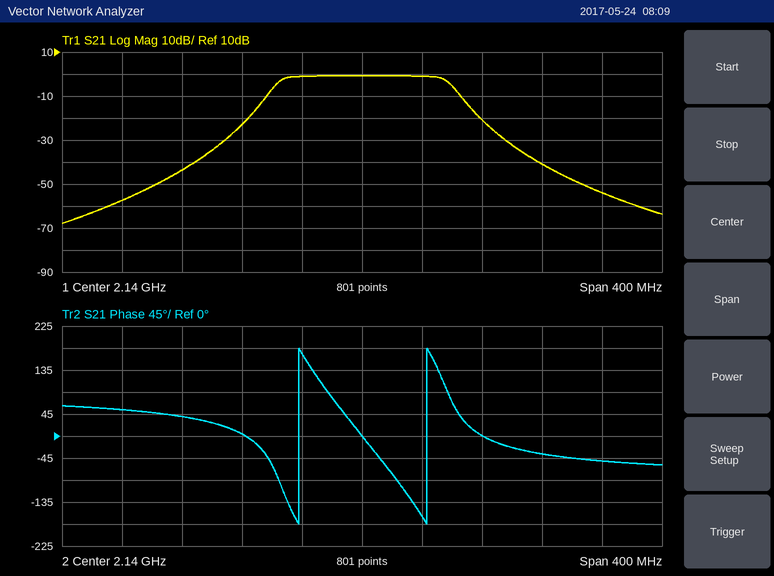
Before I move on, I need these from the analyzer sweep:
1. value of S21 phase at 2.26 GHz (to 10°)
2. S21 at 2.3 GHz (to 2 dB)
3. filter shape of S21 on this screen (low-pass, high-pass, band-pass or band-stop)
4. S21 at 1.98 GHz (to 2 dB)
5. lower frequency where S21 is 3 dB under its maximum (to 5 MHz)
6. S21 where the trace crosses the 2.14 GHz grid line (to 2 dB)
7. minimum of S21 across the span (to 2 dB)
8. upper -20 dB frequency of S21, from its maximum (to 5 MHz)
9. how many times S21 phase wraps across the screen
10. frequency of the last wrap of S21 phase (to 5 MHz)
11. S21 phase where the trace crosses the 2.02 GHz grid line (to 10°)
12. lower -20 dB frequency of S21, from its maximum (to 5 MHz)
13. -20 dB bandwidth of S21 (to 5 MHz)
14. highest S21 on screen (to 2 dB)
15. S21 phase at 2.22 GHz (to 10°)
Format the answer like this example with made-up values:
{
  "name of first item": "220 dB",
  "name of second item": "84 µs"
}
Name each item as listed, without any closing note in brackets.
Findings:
{
  "value of S21 phase at 2.26 GHz": "-40°",
  "S21 at 2.3 GHz": "-54 dB",
  "filter shape of S21 on this screen": "band-pass",
  "S21 at 1.98 GHz": "-58 dB",
  "lower frequency where S21 is 3 dB under its maximum": "2.085 GHz",
  "S21 where the trace crosses the 2.14 GHz grid line": "0 dB",
  "minimum of S21 across the span": "-68 dB",
  "upper -20 dB frequency of S21, from its maximum": "2.220 GHz",
  "how many times S21 phase wraps across the screen": "2",
  "frequency of the last wrap of S21 phase": "2.185 GHz",
  "S21 phase where the trace crosses the 2.02 GHz grid line": "40°",
  "lower -20 dB frequency of S21, from its maximum": "2.065 GHz",
  "-20 dB bandwidth of S21": "155 MHz",
  "highest S21 on screen": "0 dB",
  "S21 phase at 2.22 GHz": "0°"
}
